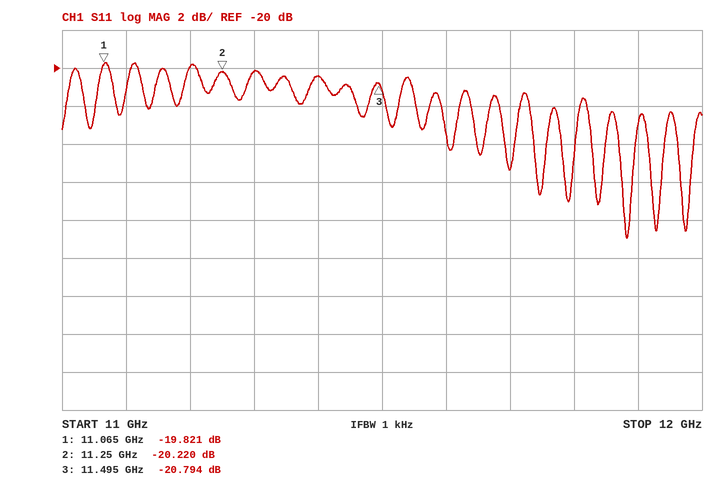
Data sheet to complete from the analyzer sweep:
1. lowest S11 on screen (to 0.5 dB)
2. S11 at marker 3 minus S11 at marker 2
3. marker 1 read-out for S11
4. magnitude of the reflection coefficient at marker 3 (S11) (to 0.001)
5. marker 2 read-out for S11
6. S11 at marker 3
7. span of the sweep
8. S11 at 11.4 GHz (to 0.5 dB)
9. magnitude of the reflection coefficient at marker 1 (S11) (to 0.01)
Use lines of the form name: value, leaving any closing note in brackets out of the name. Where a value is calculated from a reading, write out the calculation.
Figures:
lowest S11 on screen: -29.0 dB
S11 at marker 3 minus S11 at marker 2: -20.794 − (-20.22) = -0.574 dB
marker 1 read-out for S11: -19.821 dB
magnitude of the reflection coefficient at marker 3 (S11): 10^(-20.794/20) ≈ 0.091
marker 2 read-out for S11: -20.220 dB
S11 at marker 3: -20.794 dB
span of the sweep: 1 GHz
S11 at 11.4 GHz: -20.5 dB
magnitude of the reflection coefficient at marker 1 (S11): 10^(-19.821/20) ≈ 0.10
